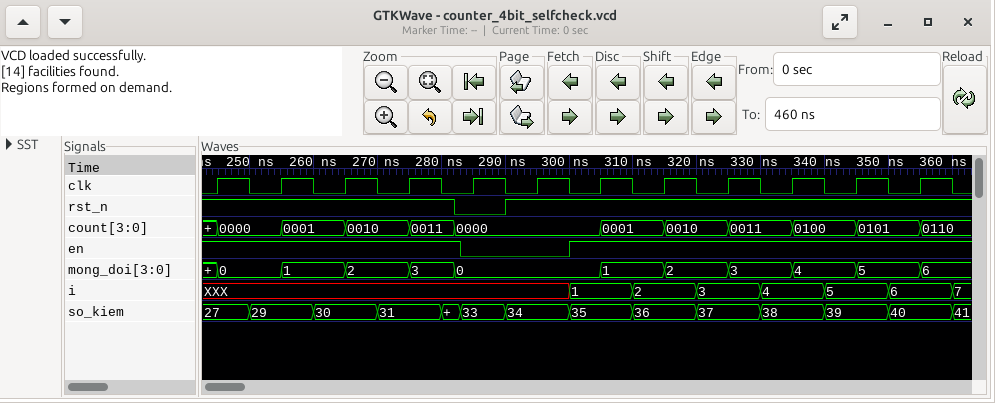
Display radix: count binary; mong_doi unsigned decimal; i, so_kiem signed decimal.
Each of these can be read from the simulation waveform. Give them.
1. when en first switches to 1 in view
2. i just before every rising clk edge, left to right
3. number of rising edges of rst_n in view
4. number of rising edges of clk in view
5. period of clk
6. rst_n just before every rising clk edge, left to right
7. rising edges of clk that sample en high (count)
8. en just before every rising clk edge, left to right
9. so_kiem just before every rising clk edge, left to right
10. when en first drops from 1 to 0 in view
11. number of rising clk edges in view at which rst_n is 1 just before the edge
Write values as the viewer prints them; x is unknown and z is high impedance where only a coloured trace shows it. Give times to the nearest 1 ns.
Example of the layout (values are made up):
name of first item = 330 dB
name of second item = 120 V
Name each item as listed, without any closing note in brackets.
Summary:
when en first switches to 1 in view = 300 ns
i just before every rising clk edge, left to right = XXX, XXX, XXX, XXX, XXX, XXX, 1, 2, 3, 4, 5, 6
number of rising edges of rst_n in view = 1
number of rising edges of clk in view = 12
period of clk = 10 ns
rst_n just before every rising clk edge, left to right = 1 1 1 1 0 1 1 1 1 1 1 1
rising edges of clk that sample en high = 10
en just before every rising clk edge, left to right = 1 1 1 1 0 0 1 1 1 1 1 1
so_kiem just before every rising clk edge, left to right = 27, 29, 30, 31, 33, 34, 35, 36, 37, 38, 39, 40
when en first drops from 1 to 0 in view = 283 ns
number of rising clk edges in view at which rst_n is 1 just before the edge = 11
